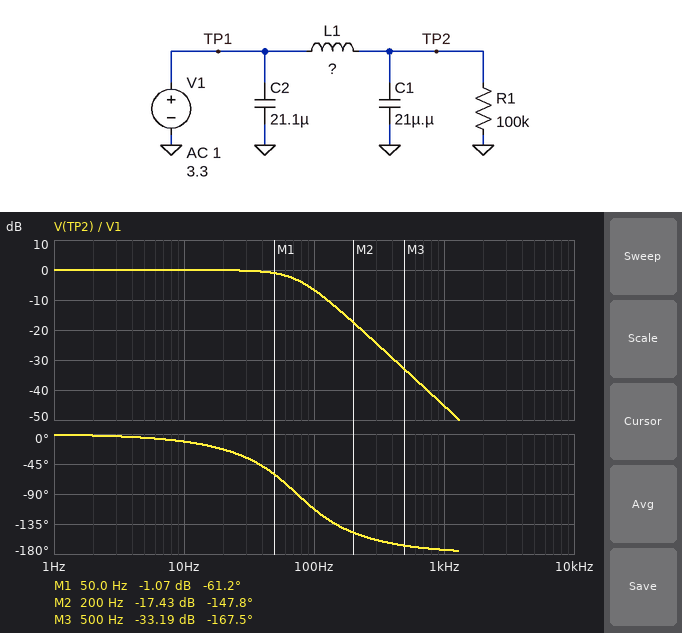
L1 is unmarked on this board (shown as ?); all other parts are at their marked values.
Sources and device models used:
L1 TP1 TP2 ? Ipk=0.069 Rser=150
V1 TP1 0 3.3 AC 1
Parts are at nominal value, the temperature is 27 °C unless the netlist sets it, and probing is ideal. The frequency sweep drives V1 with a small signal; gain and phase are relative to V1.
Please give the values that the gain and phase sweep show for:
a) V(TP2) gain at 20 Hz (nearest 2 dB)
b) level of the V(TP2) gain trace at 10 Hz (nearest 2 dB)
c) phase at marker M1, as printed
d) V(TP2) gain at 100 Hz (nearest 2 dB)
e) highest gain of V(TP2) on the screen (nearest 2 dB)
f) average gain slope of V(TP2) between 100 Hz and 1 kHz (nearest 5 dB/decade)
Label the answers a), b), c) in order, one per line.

a) 0 dB
b) 0 dB
c) -61.2 deg
d) -6 dB
e) 0 dB
f) -40 dB/decade
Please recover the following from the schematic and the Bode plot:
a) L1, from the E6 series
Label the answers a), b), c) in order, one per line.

a) 220 mH
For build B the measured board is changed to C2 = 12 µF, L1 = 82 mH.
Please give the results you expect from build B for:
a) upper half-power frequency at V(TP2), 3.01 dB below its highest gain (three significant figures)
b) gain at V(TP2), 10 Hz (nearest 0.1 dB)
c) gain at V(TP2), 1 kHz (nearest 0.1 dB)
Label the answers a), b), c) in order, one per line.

a) 60.6 Hz
b) -0.1 dB
c) -36.9 dB
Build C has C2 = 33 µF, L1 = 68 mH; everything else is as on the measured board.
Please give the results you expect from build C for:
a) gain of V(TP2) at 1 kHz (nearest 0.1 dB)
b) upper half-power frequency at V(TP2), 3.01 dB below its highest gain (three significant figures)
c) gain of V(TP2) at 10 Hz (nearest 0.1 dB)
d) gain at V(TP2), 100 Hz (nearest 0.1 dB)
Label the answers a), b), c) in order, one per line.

a) -35.4 dB
b) 58.8 Hz
c) -0.1 dB
d) -6.1 dB
